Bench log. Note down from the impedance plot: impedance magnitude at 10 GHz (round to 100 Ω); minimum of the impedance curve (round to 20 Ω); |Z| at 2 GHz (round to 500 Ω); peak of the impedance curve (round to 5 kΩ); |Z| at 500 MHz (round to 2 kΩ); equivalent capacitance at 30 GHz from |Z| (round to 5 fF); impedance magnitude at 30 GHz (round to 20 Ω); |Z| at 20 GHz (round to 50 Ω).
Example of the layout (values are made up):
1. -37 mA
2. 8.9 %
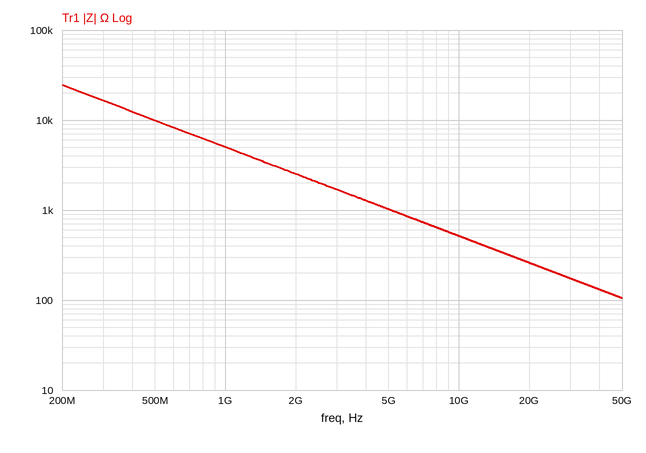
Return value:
1. 500 Ω
2. 100 Ω
3. 2.5 kΩ
4. 25 kΩ
5. 10 kΩ
6. 30 fF
7. 180 Ω
8. 250 Ω
